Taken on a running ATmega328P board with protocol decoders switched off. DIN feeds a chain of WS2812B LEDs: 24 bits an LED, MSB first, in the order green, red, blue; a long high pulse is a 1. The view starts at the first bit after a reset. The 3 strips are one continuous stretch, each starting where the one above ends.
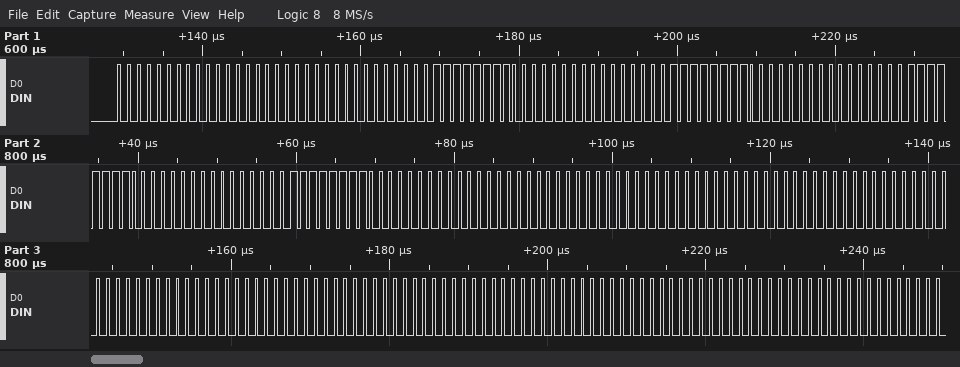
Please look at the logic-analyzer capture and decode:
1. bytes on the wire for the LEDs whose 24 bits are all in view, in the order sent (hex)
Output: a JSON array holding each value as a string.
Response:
["00 00 00 00 FF 00 00 FF 00 00 FF 00 00 FF 00 00 00 00 00 00 00 00 00 00 00 00 00 00 00 00"]
